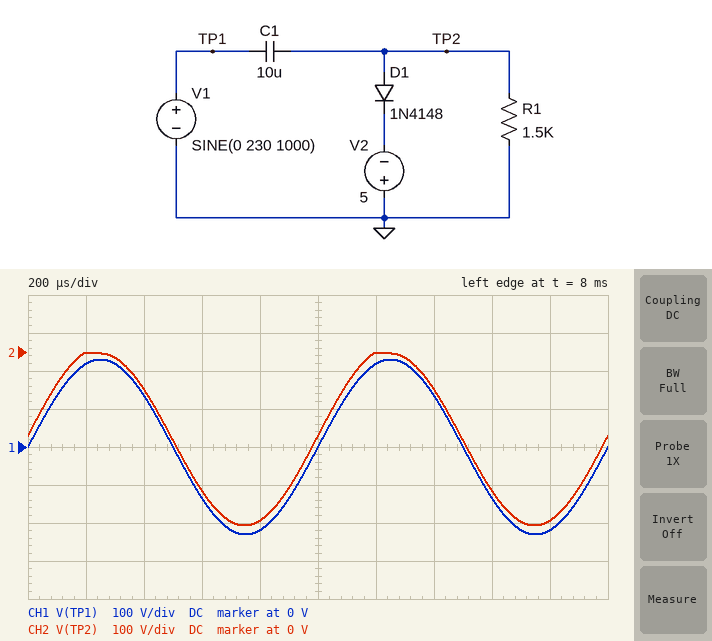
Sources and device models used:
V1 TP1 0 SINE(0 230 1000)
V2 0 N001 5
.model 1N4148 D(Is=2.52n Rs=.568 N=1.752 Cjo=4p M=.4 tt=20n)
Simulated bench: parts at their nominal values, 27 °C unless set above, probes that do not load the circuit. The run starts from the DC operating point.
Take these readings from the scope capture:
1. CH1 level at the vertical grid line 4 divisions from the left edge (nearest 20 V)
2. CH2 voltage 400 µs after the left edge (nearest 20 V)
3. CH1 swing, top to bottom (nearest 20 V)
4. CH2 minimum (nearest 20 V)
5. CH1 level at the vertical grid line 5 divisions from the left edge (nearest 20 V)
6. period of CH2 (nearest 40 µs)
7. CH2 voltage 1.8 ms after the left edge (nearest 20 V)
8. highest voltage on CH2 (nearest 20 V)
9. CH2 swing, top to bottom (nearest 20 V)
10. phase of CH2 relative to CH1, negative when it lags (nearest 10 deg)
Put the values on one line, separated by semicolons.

-220 V; -100 V; 460 V; -460 V; 0 V; 1.00 ms; -440 V; 0 V; 460 V; 0 deg
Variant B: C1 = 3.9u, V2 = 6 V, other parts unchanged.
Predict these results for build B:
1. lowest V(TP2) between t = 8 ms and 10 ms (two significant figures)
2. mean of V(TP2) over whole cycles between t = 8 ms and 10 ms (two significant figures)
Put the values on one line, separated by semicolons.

-450 V; -220 V
